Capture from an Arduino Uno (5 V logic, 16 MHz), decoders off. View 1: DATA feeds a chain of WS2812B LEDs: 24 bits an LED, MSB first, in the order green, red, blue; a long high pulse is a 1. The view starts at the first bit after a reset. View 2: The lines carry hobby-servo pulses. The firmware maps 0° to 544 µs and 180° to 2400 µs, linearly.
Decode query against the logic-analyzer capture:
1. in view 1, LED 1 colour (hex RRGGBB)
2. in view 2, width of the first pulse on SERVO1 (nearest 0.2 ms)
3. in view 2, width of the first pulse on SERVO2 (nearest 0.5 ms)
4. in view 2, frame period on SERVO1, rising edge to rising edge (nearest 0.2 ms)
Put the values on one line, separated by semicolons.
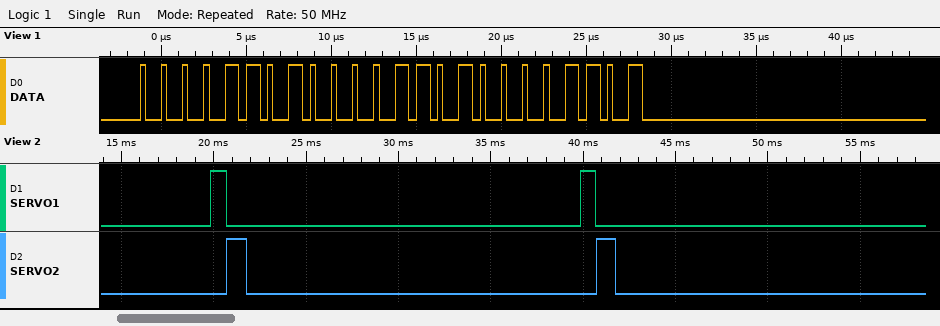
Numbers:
#0D0D0D; 0.8 ms; 1.0 ms; 20.0 ms
